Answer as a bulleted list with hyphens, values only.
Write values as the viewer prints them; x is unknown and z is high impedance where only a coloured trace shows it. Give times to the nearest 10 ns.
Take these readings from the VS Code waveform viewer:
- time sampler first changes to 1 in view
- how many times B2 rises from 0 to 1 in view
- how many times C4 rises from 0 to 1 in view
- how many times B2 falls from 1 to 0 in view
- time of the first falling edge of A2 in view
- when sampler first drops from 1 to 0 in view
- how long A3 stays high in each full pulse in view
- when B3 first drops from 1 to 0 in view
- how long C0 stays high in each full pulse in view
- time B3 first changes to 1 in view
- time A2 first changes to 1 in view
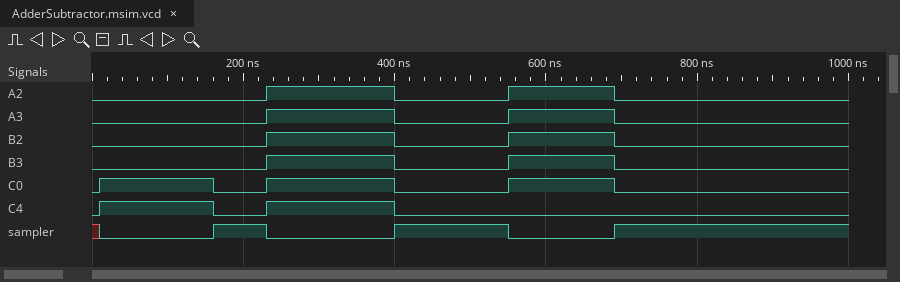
- 160 ns
- 2
- 2
- 2
- 400 ns
- 230 ns
- 170 ns, 140 ns
- 400 ns
- 150 ns, 170 ns, 140 ns
- 230 ns
- 230 ns
